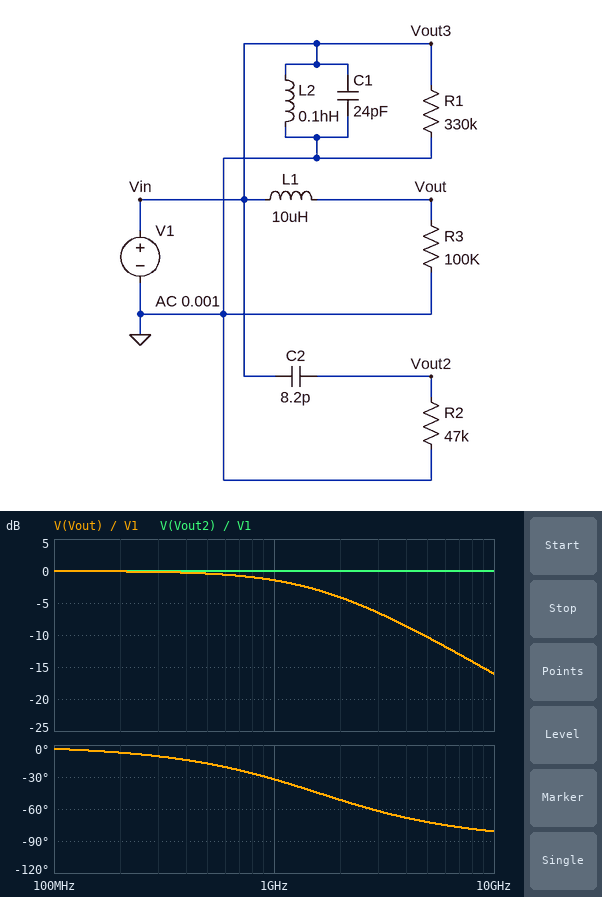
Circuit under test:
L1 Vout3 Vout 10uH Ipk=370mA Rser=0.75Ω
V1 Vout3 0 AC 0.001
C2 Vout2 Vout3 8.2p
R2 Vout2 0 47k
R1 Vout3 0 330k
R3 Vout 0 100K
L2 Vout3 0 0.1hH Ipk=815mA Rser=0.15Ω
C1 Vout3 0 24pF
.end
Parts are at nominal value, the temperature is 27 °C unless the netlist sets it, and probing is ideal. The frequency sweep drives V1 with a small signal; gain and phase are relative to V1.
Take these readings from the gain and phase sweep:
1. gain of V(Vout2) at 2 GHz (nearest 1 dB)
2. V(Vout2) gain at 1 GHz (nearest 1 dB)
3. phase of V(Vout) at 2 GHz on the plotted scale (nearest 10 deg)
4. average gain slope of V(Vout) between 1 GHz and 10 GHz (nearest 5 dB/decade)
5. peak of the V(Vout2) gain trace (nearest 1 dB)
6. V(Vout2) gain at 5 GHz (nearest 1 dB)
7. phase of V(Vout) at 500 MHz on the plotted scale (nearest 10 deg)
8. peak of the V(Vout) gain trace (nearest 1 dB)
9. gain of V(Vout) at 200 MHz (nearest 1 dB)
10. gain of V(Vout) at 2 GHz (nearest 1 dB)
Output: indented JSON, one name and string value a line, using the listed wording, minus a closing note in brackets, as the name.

{
  "gain of V(Vout2) at 2 GHz": "0 dB",
  "V(Vout2) gain at 1 GHz": "0 dB",
  "phase of V(Vout) at 2 GHz on the plotted scale": "-50 deg",
  "average gain slope of V(Vout) between 1 GHz and 10 GHz": "-15 dB/decade",
  "peak of the V(Vout2) gain trace": "0 dB",
  "V(Vout2) gain at 5 GHz": "0 dB",
  "phase of V(Vout) at 500 MHz on the plotted scale": "-20 deg",
  "peak of the V(Vout) gain trace": "0 dB",
  "gain of V(Vout) at 200 MHz": "0 dB",
  "gain of V(Vout) at 2 GHz": "-4 dB"
}
